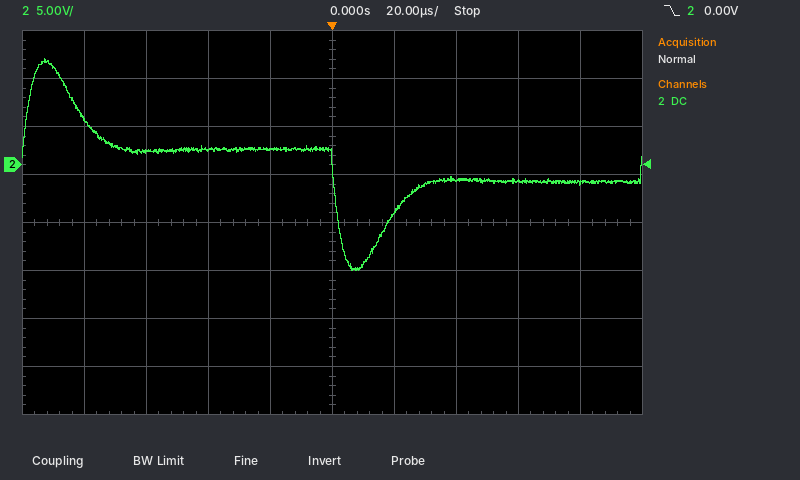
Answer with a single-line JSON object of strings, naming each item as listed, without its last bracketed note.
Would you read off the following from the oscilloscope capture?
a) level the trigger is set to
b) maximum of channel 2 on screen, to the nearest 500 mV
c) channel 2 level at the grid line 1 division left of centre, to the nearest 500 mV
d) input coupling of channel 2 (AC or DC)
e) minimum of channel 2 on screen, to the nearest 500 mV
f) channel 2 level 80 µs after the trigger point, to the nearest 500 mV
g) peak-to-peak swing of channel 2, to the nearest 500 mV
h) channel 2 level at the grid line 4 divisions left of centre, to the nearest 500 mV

{"level the trigger is set to": "0.00 V", "maximum of channel 2 on screen, to the nearest 500 mV": "11.0 V", "channel 2 level at the grid line 1 division left of centre, to the nearest 500 mV": "1.5 V", "input coupling of channel 2": "DC", "minimum of channel 2 on screen, to the nearest 500 mV": "-11.0 V", "channel 2 level 80 µs after the trigger point, to the nearest 500 mV": "-2.0 V", "peak-to-peak swing of channel 2, to the nearest 500 mV": "22.0 V", "channel 2 level at the grid line 4 divisions left of centre, to the nearest 500 mV": "5.0 V"}
